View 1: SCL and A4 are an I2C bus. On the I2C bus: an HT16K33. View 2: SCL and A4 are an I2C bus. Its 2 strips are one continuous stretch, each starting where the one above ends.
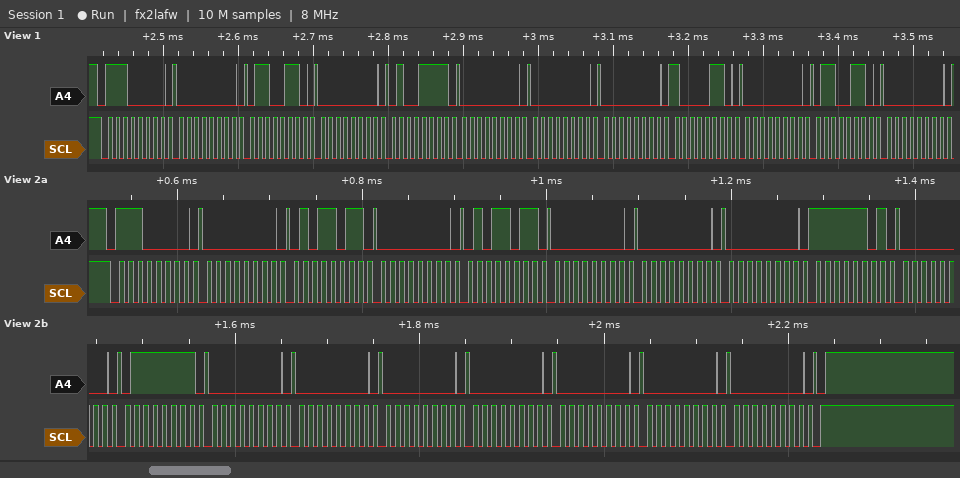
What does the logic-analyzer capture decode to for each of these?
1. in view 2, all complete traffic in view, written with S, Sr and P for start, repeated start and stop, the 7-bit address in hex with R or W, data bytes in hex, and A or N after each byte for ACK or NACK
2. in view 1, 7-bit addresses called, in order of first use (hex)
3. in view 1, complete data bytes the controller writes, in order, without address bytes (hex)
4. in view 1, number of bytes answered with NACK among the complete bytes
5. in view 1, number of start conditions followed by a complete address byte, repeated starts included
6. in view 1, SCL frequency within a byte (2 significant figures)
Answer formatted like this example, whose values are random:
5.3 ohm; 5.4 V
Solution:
S 70W A 00 A 5B A 00 A 5B A 00 A 00 A 00 A FD A 00 A 7F A 00 A 00 A 00 A 00 A 00 A 00 A 00 A P; 0x70; 00 66 00 4F 00 00 00 86 00 66 00; 0; 1; 100 kHz
